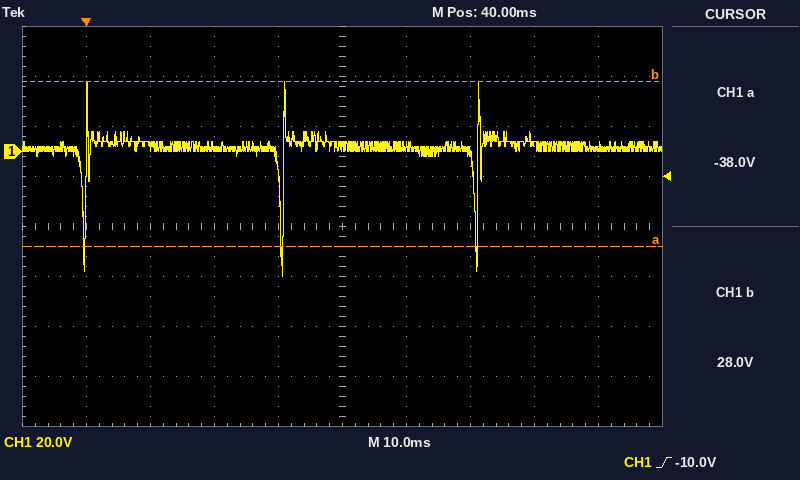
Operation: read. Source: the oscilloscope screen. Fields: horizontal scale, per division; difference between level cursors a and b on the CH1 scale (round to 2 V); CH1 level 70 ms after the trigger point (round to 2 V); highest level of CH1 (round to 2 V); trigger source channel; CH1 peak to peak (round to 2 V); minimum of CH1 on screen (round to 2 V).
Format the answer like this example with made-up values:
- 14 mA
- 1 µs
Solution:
- 10 ms
- 66 V
- 2 V
- 28 V
- CH1
- 78 V
- -50 V
